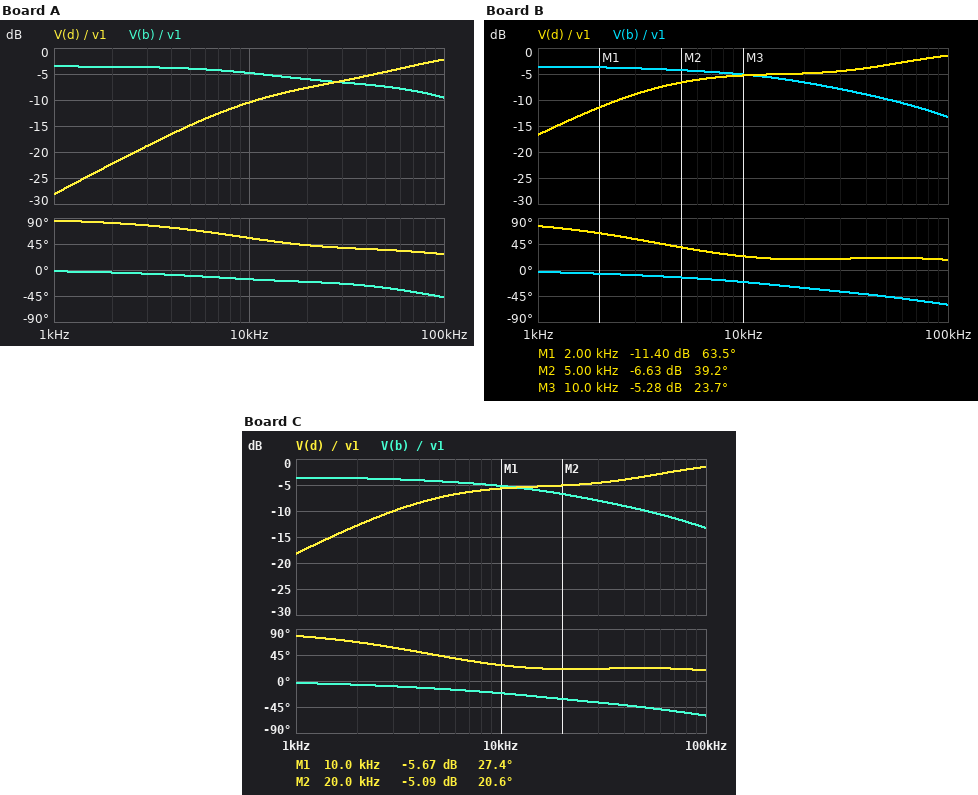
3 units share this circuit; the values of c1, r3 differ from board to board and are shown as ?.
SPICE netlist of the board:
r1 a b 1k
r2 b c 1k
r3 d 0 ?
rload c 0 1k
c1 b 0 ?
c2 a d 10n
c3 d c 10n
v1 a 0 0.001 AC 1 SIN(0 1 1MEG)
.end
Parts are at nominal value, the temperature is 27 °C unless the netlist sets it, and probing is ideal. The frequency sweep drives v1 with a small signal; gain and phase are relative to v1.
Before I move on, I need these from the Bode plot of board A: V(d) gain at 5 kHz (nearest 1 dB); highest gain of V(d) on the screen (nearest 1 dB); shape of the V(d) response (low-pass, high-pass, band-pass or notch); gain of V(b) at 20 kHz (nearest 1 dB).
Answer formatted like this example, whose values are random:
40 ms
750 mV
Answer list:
-15 dB
-2 dB
high-pass
-6 dB
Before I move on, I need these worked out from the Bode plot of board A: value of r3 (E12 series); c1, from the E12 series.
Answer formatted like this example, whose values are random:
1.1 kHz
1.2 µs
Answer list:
470 Ω
6.8 nF
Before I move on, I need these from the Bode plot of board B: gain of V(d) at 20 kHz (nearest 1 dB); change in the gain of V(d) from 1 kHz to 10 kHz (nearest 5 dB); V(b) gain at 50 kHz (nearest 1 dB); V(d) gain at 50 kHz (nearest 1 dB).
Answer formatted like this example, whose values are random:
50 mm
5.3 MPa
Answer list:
-5 dB
10 dB
-10 dB
-3 dB
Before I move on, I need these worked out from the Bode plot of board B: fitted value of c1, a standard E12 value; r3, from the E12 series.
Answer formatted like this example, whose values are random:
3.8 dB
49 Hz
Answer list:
12 nF
1.8 kΩ
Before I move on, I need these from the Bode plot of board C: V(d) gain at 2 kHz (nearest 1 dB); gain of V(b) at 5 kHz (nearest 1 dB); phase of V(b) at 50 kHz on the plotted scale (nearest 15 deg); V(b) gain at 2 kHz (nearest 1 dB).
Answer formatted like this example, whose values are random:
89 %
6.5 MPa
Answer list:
-13 dB
-4 dB
-45 deg
-4 dB
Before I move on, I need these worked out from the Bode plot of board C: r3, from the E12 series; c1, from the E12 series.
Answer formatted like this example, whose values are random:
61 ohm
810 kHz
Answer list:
1.5 kΩ
12 nF
